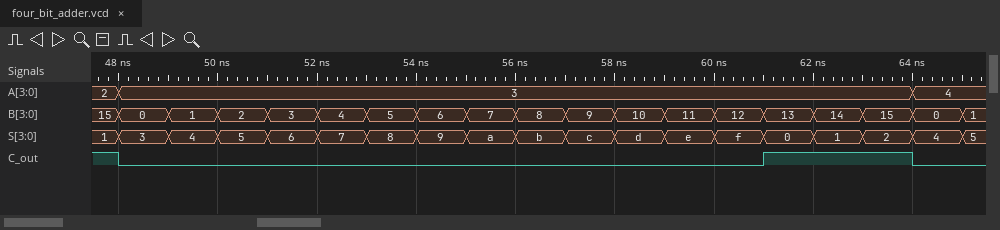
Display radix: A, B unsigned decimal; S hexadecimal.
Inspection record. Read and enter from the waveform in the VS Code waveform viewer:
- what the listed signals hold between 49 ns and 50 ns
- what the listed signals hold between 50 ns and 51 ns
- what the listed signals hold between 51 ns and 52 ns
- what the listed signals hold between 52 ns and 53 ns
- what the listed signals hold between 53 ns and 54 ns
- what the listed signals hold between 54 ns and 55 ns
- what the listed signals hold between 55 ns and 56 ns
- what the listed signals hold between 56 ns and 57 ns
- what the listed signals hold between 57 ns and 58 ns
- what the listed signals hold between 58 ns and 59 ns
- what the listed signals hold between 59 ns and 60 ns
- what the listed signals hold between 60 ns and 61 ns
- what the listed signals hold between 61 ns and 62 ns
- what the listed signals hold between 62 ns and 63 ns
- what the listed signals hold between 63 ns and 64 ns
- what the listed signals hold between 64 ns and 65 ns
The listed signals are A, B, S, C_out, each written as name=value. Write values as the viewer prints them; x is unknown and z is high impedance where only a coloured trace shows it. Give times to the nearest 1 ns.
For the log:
A=3, B=1, S=4, C_out=0
A=3, B=2, S=5, C_out=0
A=3, B=3, S=6, C_out=0
A=3, B=4, S=7, C_out=0
A=3, B=5, S=8, C_out=0
A=3, B=6, S=9, C_out=0
A=3, B=7, S=a, C_out=0
A=3, B=8, S=b, C_out=0
A=3, B=9, S=c, C_out=0
A=3, B=10, S=d, C_out=0
A=3, B=11, S=e, C_out=0
A=3, B=12, S=f, C_out=0
A=3, B=13, S=0, C_out=1
A=3, B=14, S=1, C_out=1
A=3, B=15, S=2, C_out=1
A=4, B=0, S=4, C_out=0
